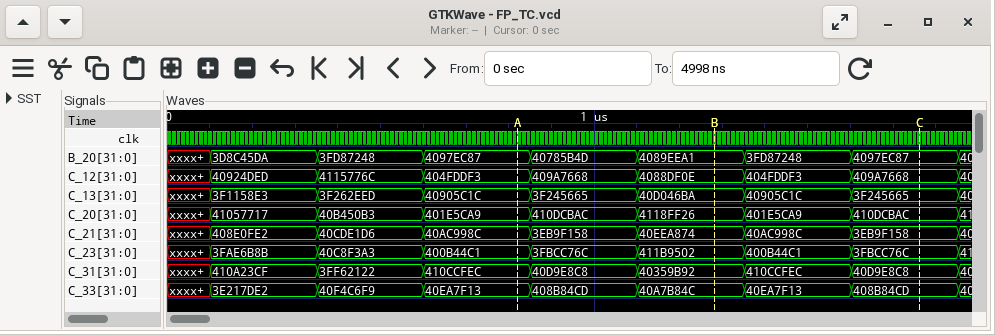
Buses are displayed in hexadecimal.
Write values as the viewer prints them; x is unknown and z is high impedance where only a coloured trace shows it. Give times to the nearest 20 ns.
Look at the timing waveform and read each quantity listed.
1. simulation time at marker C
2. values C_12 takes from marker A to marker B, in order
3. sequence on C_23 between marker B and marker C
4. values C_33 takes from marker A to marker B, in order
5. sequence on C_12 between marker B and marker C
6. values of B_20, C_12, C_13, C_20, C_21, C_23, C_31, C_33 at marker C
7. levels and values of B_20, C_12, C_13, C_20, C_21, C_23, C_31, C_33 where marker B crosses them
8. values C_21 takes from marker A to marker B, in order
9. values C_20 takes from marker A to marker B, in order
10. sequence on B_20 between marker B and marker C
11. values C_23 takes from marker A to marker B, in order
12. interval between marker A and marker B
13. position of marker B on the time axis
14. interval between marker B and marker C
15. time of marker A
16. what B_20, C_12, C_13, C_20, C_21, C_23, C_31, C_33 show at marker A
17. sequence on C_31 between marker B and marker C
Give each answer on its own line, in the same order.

1760 ns
404FDDF3, 409A7668, 4088DF0E
411B9502, 400B44C1, 3FBCC76C
40EA7F13, 408B84CD, 40A7B84C
4088DF0E, 404FDDF3, 409A7668
B_20=4097EC87, C_12=409A7668, C_13=3F245665, C_20=410DCBAC, C_21=3EB9F158, C_23=3FBCC76C, C_31=40D9E8C8, C_33=408B84CD
B_20=4089EEA1, C_12=4088DF0E, C_13=40D046BA, C_20=4118FF26, C_21=40EEA874, C_23=411B9502, C_31=40359B92, C_33=40A7B84C
40AC998C, 3EB9F158, 40EEA874
401E5CA9, 410DCBAC, 4118FF26
4089EEA1, 3FD87248, 4097EC87
400B44C1, 3FBCC76C, 411B9502
460 ns
1280 ns
480 ns
820 ns
B_20=4097EC87, C_12=404FDDF3, C_13=40905C1C, C_20=401E5CA9, C_21=40AC998C, C_23=400B44C1, C_31=410CCFEC, C_33=40EA7F13
40359B92, 410CCFEC, 40D9E8C8
